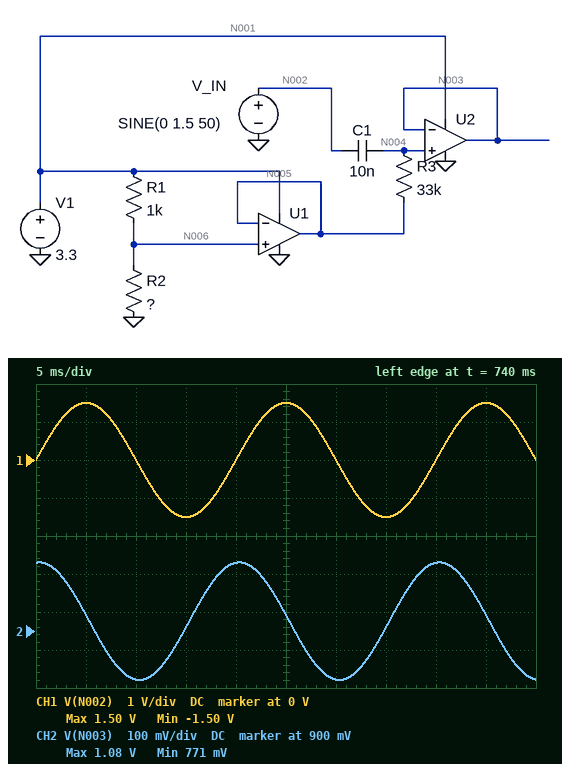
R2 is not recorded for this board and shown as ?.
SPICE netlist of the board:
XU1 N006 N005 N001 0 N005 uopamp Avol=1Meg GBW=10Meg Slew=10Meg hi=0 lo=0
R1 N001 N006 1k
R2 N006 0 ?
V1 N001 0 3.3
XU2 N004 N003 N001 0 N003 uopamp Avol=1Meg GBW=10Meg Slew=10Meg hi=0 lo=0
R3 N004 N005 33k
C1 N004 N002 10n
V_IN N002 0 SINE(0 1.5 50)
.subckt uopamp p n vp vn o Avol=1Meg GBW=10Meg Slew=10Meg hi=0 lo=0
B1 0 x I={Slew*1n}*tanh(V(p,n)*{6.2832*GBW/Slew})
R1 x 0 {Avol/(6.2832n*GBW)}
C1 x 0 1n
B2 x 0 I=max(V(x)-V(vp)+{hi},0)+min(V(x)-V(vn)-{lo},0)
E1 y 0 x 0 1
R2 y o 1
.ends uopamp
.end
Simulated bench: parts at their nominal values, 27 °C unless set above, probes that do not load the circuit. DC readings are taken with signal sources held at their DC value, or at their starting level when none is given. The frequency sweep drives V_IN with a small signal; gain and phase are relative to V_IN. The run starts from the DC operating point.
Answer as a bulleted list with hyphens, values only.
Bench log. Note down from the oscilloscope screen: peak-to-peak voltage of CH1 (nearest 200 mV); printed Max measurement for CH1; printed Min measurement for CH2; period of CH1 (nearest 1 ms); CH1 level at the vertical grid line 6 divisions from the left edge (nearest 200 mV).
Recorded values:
- 3.0 V
- 1.50 V
- 771 mV
- 20 ms
- 0 V
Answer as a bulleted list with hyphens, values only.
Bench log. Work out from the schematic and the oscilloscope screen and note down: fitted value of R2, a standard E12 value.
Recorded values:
- 390 Ω
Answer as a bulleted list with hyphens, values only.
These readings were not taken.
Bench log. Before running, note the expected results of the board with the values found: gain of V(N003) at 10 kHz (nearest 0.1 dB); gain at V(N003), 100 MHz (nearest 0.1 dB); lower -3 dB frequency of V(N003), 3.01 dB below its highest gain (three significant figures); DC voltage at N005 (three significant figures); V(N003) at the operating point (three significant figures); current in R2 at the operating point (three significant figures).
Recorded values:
- 0 dB
- -20.0 dB
- 482 Hz
- 926 mV
- 926 mV
- 2.37 mA
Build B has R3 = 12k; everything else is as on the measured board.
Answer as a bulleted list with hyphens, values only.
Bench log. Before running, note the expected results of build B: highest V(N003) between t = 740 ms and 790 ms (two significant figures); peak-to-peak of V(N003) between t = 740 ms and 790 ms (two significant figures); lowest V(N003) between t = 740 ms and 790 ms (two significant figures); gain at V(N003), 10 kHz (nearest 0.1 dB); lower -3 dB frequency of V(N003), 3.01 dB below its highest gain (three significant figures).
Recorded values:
- 980 mV
- 110 mV
- 870 mV
- -0.1 dB
- 1.33 kHz
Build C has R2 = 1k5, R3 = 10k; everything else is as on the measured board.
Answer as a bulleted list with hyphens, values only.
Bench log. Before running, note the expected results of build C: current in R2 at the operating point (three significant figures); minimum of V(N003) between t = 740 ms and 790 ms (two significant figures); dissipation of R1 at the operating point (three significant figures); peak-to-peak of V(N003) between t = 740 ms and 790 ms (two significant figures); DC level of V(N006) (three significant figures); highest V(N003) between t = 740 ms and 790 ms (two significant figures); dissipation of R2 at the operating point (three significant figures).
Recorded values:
- 1.32 mA
- 1.9 V
- 1.74 mW
- 94 mV
- 1.98 V
- 2.0 V
- 2.61 mW
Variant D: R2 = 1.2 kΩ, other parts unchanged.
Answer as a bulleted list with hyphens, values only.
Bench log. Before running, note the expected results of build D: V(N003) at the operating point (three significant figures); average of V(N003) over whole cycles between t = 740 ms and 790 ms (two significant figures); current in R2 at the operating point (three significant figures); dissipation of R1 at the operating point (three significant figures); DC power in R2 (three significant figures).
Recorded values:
- 1.80 V
- 1.8 V
- 1.50 mA
- 2.25 mW
- 2.70 mW
